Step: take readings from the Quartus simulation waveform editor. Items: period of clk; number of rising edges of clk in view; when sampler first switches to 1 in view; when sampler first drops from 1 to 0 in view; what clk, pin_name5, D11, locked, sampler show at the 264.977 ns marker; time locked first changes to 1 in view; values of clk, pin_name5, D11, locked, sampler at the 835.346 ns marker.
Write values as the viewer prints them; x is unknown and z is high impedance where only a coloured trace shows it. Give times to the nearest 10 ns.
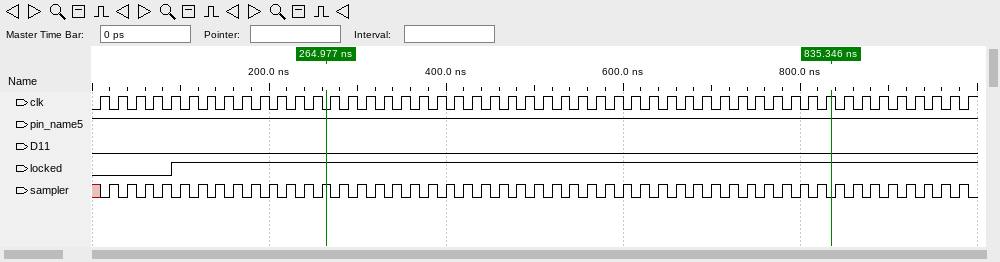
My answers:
20 ns
50
20 ns
30 ns
clk=0, pin_name5=1, D11=0, locked=1, sampler=1
90 ns
clk=1, pin_name5=1, D11=0, locked=1, sampler=0
